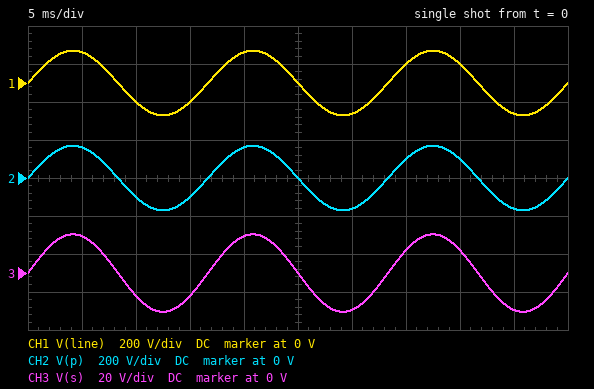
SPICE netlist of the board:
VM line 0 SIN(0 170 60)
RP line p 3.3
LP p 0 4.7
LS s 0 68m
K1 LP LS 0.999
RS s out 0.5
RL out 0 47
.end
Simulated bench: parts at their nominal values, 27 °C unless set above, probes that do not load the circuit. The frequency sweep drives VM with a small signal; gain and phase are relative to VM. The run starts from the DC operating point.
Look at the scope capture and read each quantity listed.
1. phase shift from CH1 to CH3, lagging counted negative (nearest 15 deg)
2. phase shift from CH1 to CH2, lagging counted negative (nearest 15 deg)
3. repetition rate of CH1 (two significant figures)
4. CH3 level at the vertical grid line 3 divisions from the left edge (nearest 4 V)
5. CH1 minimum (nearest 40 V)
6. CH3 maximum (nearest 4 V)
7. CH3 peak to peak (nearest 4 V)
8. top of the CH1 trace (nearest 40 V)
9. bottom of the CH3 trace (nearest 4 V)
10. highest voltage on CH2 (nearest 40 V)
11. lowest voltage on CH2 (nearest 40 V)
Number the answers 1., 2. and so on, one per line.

1. 0 deg
2. 0 deg
3. 60 Hz
4. -12 V
5. -160 V
6. 20 V
7. 40 V
8. 160 V
9. -20 V
10. 160 V
11. -160 V
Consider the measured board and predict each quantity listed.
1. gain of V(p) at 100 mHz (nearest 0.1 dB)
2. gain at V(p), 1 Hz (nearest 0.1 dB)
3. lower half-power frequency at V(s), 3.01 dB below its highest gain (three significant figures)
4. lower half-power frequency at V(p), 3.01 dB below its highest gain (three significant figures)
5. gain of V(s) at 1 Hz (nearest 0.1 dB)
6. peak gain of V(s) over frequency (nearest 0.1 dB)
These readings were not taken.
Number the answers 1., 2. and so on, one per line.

1. -3.5 dB
2. -0.1 dB
3. 112 mHz
4. 112 mHz
5. -18.5 dB
6. -18.4 dB
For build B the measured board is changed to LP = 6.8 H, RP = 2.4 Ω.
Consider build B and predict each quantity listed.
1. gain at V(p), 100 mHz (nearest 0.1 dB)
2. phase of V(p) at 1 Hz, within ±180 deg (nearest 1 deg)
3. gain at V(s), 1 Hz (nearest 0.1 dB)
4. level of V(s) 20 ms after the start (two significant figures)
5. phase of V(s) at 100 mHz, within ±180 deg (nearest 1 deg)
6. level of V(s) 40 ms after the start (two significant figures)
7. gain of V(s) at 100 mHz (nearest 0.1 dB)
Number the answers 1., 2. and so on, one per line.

1. -1.2 dB
2. 3 deg
3. -20.0 dB
4. 16 V
5. 29 deg
6. 10 V
7. -21.2 dB
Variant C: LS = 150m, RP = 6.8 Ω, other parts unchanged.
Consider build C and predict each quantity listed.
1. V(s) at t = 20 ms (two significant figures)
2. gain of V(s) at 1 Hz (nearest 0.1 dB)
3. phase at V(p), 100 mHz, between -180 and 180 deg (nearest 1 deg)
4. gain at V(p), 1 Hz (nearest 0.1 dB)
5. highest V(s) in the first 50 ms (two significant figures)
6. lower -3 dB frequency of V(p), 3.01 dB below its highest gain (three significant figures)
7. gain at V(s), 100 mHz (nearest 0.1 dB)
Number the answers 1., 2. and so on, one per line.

1. 29 V
2. -15.2 dB
3. 66 deg
4. -0.3 dB
5. 30 V
6. 229 mHz
7. -23.0 dB
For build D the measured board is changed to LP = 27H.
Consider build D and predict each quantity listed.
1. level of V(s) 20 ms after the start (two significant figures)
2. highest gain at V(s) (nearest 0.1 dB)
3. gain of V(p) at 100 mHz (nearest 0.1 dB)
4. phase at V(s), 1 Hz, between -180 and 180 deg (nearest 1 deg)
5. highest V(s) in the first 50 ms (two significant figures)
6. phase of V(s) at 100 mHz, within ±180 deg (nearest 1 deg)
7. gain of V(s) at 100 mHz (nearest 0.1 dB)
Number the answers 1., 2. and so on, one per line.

1. 8.1 V
2. -26.0 dB
3. -0.2 dB
4. 1 deg
5. 8.5 V
6. 11 deg
7. -26.2 dB
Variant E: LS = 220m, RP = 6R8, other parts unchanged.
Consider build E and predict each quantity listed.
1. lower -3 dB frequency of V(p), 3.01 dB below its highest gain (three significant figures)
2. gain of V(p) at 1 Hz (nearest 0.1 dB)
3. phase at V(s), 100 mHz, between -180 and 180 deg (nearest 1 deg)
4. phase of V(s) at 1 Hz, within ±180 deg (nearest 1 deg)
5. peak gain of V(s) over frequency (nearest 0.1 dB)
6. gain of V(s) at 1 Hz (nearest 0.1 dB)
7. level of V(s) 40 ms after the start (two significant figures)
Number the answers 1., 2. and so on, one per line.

1. 229 mHz
2. -0.3 dB
3. 66 deg
4. 13 deg
5. -13.4 dB
6. -13.6 dB
7. 21 V
